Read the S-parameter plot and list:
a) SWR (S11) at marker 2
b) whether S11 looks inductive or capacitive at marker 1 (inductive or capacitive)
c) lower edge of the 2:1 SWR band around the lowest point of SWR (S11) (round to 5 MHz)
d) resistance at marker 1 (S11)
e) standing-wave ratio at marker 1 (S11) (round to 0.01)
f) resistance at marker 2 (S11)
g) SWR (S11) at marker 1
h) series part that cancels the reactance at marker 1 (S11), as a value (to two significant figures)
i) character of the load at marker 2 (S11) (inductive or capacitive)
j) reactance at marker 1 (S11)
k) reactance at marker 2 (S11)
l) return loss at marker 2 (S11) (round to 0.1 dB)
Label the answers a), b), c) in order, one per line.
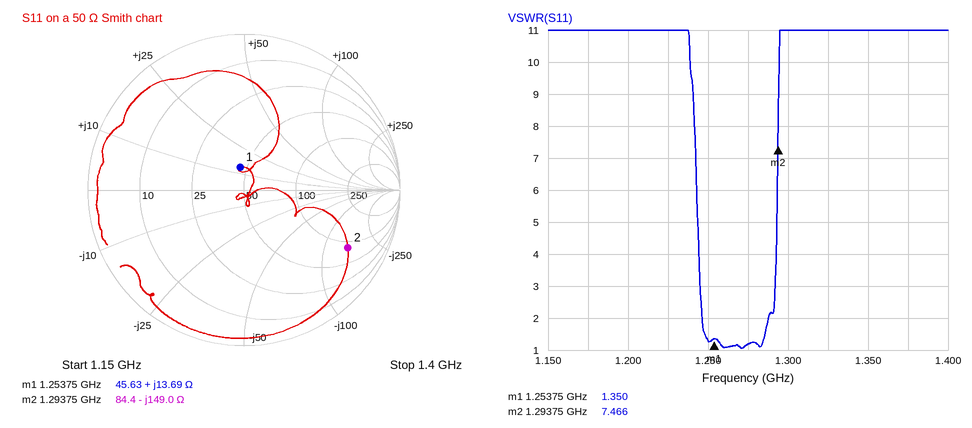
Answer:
a) 7.466
b) inductive
c) 1.245 GHz
d) 45.63 Ω
e) 1.35
f) 84.4 Ω
g) 1.350
h) 9.3 pF
i) capacitive
j) +13.69 Ω
k) -149.0 Ω
l) 2.4 dB
